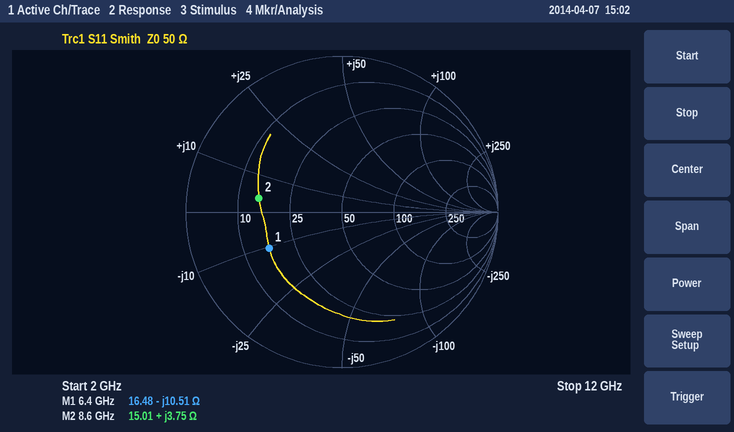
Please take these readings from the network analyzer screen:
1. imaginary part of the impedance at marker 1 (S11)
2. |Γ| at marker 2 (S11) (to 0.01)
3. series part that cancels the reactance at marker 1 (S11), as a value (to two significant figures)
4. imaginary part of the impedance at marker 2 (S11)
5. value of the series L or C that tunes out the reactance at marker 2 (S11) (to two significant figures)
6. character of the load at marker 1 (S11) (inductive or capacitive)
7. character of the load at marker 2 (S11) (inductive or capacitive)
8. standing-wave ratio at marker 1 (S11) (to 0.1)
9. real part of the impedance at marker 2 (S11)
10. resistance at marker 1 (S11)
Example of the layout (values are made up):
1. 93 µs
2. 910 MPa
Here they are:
1. -10.51 Ω
2. 0.54
3. 260 pH
4. +3.75 Ω
5. 4.9 pF
6. capacitive
7. inductive
8. 3.2
9. 15.01 Ω
10. 16.48 Ω
